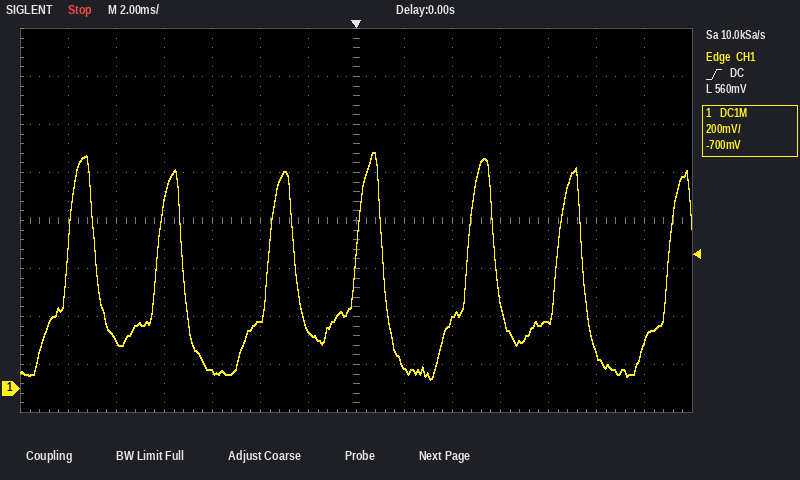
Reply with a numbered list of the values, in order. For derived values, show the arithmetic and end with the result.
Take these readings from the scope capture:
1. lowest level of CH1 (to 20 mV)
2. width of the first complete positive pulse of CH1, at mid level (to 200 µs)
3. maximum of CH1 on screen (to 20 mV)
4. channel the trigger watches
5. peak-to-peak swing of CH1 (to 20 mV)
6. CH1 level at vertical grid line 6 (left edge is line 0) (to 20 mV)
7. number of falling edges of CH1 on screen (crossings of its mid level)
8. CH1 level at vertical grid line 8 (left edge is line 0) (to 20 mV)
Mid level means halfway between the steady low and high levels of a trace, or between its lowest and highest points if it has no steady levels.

1. 40 mV
2. 1.2 ms
3. 980 mV
4. CH1
5. 980 mV − (40 mV) = 940 mV
6. 240 mV
7. 6
8. 80 mV
